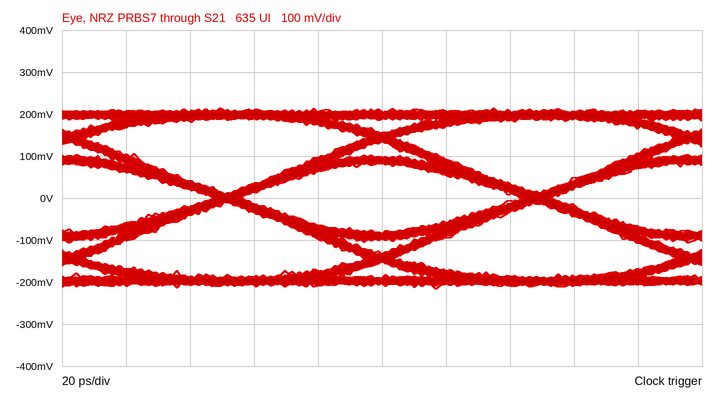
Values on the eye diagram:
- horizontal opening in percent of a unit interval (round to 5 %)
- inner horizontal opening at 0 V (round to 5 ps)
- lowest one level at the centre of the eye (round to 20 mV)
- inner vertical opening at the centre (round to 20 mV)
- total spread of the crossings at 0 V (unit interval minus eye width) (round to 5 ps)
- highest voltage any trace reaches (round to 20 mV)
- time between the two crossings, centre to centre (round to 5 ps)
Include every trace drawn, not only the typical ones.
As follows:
90 %
85 ps
80 mV
160 mV
10 ps
220 mV
95 ps
